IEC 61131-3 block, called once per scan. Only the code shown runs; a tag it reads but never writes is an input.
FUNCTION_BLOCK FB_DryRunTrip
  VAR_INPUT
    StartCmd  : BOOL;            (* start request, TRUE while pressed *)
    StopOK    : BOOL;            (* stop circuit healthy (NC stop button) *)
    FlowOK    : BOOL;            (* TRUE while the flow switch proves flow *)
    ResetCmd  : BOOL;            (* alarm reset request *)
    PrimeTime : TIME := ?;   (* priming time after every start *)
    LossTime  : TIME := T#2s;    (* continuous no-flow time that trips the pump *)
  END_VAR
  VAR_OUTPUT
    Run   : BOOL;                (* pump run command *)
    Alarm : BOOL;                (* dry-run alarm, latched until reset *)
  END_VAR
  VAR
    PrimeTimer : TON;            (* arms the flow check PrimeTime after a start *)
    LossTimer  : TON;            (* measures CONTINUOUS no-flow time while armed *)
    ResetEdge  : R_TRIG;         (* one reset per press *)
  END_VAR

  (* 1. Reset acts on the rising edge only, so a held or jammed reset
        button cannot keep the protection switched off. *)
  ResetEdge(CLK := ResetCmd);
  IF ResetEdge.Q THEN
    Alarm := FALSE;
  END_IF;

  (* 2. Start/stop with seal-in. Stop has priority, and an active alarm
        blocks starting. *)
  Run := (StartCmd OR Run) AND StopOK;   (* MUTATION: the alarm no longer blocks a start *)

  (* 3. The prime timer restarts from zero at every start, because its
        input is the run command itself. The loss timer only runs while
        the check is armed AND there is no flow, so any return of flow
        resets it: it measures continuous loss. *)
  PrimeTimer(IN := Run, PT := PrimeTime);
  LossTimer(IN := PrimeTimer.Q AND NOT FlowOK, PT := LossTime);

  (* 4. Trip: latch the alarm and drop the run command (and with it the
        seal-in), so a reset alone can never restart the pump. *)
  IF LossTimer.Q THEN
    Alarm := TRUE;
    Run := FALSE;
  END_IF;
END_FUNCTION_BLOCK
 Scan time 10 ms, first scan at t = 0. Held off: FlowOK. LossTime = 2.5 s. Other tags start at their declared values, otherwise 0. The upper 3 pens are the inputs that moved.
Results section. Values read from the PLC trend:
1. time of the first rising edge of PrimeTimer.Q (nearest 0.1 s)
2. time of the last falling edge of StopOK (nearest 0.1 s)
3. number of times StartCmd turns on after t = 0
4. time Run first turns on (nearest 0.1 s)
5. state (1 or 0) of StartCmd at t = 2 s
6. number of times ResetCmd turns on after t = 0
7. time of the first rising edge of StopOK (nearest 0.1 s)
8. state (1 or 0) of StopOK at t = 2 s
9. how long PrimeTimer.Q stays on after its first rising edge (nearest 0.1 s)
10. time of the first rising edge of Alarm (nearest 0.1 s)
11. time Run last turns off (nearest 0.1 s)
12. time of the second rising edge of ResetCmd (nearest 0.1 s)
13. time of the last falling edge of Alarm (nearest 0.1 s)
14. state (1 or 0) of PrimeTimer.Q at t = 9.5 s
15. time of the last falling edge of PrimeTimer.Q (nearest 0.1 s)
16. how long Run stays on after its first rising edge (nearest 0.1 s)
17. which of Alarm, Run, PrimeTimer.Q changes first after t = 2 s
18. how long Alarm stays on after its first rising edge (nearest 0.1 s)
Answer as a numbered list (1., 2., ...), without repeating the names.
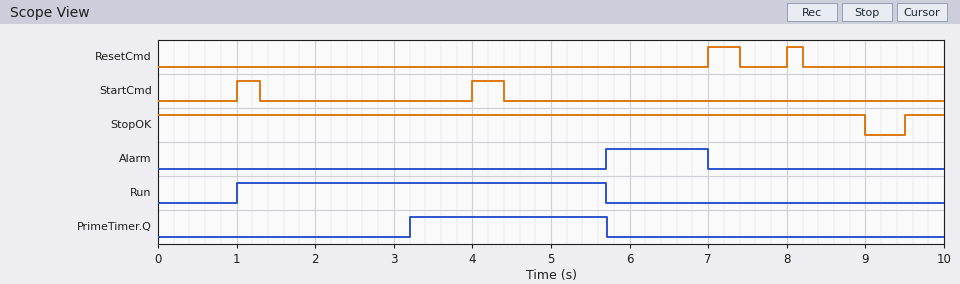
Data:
1. 3.2 s
2. 9.0 s
3. 2
4. 1.0 s
5. 0
6. 2
7. 9.5 s
8. 1
9. 2.5 s
10. 5.7 s
11. 5.7 s
12. 8.0 s
13. 7.0 s
14. 0
15. 5.7 s
16. 4.7 s
17. PrimeTimer.Q
18. 1.3 s
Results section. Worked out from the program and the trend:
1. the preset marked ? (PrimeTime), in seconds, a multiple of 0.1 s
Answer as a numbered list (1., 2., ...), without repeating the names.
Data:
1. 2.2 s
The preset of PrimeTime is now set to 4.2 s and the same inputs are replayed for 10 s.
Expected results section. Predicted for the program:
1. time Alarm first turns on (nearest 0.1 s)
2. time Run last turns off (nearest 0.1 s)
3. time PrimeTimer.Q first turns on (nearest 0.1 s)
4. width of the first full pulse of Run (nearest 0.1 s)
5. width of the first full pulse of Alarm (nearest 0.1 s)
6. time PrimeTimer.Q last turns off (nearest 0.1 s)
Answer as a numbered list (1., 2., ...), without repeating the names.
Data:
1. 7.7 s
2. 7.7 s
3. 5.2 s
4. 6.7 s
5. 0.3 s
6. 7.7 s
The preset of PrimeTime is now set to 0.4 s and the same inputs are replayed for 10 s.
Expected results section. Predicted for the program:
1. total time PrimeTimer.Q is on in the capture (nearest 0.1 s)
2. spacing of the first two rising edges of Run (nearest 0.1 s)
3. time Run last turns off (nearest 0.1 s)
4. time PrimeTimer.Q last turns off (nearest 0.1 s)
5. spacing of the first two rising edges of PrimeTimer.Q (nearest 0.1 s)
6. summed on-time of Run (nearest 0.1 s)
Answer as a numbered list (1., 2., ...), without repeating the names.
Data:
1. 5.0 s
2. 3.0 s
3. 6.9 s
4. 6.9 s
5. 3.0 s
6. 5.8 s
